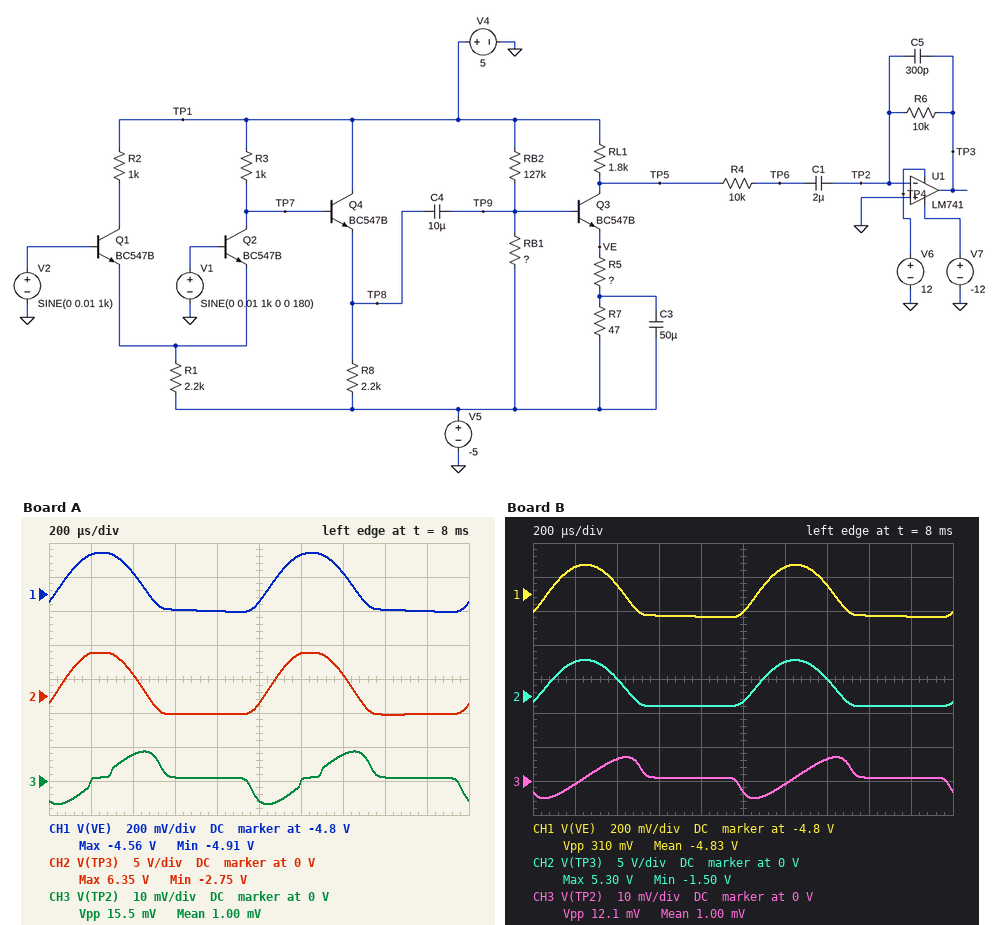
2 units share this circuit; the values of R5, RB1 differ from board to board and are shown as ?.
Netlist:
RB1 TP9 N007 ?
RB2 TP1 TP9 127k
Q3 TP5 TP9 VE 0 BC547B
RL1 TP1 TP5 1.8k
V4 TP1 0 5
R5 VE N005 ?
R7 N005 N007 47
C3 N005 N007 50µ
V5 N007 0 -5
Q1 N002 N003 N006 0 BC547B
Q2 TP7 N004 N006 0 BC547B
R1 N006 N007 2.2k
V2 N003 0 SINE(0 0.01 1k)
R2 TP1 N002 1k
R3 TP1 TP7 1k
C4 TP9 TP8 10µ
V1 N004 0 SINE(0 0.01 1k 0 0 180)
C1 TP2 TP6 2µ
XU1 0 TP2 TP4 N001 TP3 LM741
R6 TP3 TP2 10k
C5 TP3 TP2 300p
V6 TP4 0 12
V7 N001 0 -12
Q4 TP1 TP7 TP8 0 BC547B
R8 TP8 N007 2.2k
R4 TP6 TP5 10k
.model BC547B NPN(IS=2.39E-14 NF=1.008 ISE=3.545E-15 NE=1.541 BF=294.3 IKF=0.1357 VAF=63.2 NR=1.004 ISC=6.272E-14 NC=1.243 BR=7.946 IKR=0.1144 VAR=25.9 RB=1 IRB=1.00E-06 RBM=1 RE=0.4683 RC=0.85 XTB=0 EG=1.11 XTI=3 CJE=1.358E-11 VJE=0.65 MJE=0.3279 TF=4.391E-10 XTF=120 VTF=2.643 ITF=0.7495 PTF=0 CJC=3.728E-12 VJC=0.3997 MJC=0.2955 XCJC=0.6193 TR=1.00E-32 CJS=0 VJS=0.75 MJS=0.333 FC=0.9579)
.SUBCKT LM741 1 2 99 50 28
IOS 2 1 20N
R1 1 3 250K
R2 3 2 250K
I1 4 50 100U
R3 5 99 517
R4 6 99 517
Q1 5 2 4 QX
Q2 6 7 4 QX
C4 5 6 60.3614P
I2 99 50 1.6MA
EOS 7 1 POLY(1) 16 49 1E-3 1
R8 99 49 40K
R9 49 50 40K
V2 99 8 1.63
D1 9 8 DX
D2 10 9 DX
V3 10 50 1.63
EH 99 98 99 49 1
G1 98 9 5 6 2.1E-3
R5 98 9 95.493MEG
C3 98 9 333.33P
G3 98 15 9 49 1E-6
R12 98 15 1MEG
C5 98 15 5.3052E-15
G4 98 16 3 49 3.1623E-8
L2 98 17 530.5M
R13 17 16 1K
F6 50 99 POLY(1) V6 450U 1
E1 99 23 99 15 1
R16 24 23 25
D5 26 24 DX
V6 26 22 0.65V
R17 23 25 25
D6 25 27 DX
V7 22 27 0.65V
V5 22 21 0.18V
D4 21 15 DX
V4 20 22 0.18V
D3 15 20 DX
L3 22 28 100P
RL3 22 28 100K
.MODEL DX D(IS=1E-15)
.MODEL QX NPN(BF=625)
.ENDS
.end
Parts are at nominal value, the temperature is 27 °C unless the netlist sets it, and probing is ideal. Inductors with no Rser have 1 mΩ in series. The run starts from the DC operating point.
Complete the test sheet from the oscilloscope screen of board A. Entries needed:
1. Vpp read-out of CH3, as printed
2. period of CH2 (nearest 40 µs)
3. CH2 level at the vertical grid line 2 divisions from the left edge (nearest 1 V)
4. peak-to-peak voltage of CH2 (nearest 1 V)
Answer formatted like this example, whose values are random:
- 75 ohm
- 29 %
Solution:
- 15.5 mV
- 1.00 ms
- 3 V
- 9 V
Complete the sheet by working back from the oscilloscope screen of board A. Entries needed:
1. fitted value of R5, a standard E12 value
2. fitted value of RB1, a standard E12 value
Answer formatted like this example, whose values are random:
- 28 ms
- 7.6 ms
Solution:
- 56 Ω
- 12 kΩ
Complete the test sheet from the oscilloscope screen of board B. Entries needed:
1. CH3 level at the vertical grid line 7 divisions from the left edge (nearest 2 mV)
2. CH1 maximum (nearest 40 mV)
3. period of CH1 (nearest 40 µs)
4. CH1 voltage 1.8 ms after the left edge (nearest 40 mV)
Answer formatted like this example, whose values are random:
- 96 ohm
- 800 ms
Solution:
- 6 mV
- -4.64 V
- 1.00 ms
- -4.92 V
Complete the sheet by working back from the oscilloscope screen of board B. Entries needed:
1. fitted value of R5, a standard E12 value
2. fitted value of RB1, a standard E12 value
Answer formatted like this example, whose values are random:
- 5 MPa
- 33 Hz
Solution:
- 68 Ω
- 10 kΩ
